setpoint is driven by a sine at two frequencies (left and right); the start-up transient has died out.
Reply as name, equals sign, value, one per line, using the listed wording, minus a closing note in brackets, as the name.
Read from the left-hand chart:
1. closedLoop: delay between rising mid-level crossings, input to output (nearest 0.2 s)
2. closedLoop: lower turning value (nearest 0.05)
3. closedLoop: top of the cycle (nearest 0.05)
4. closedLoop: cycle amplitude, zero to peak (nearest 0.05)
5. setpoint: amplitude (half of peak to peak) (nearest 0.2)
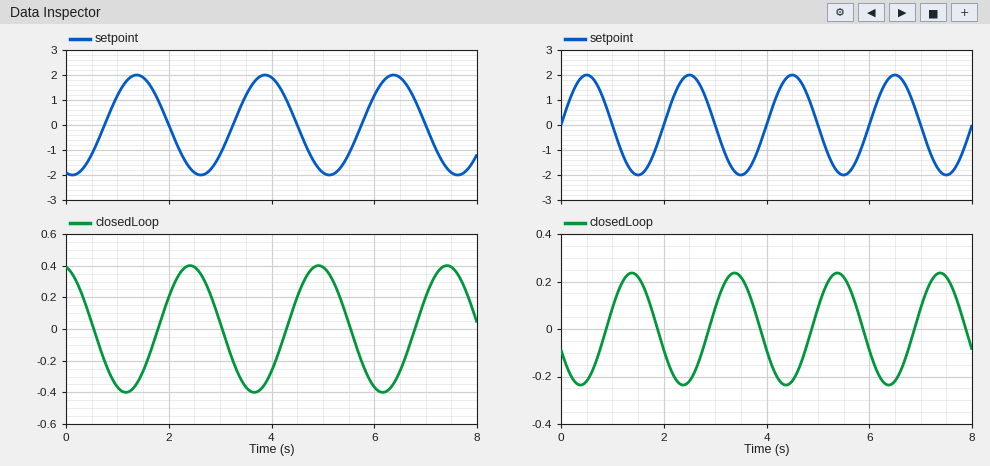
closedLoop: delay between rising mid-level crossings, input to output = 1.0 s
closedLoop: lower turning value = -0.40
closedLoop: top of the cycle = 0.40
closedLoop: cycle amplitude, zero to peak = 0.40
setpoint: amplitude (half of peak to peak) = 2.0
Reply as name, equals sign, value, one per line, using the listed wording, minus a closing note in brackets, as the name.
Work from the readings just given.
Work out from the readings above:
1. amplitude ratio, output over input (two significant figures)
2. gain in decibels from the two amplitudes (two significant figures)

amplitude ratio, output over input = 0.20
gain in decibels from the two amplitudes = -14 dB
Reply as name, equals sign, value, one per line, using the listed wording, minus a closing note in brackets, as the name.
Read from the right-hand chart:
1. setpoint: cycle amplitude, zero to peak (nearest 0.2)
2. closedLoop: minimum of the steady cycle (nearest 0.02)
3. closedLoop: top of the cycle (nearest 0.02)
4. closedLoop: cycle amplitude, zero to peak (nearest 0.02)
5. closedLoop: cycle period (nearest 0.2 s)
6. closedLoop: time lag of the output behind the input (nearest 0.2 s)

setpoint: cycle amplitude, zero to peak = 2.0
closedLoop: minimum of the steady cycle = -0.24
closedLoop: top of the cycle = 0.24
closedLoop: cycle amplitude, zero to peak = 0.24
closedLoop: cycle period = 2.0 s
closedLoop: time lag of the output behind the input = 0.8 s
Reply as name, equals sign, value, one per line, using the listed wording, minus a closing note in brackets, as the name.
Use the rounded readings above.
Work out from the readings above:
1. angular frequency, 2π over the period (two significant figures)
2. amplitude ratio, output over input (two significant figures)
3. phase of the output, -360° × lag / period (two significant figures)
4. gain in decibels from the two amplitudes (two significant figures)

angular frequency, 2π over the period = 3.1 rad/s
amplitude ratio, output over input = 0.12
phase of the output, -360° × lag / period = -140°
gain in decibels from the two amplitudes = -18 dB
